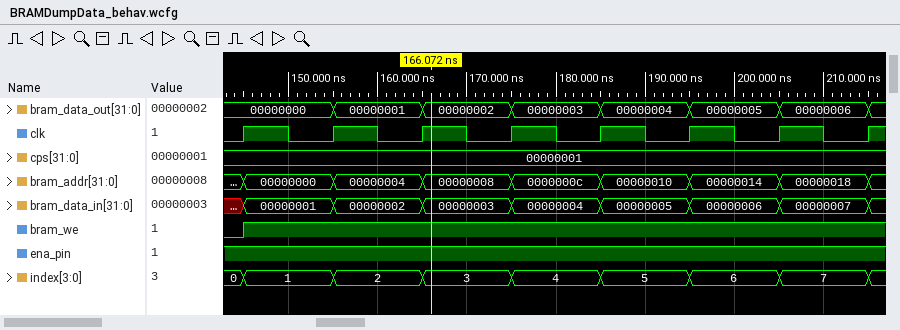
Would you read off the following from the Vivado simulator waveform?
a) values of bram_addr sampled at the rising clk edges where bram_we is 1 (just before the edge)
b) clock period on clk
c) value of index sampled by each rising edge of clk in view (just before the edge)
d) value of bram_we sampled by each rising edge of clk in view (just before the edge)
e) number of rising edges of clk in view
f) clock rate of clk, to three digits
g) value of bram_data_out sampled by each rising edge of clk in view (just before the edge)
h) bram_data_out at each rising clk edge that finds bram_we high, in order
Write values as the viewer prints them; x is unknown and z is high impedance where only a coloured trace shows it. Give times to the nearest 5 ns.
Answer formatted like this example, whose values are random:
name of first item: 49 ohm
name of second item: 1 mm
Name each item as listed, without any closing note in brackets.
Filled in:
values of bram_addr sampled at the rising clk edges where bram_we is 1: 00000000, 00000004, 00000008, 0000000c, 00000010, 00000014, 00000018
clock period on clk: 10 ns
value of index sampled by each rising edge of clk in view: 0, 1, 2, 3, 4, 5, 6, 7
value of bram_we sampled by each rising edge of clk in view: 0 1 1 1 1 1 1 1
number of rising edges of clk in view: 8
clock rate of clk, to three digits: 100 MHz
value of bram_data_out sampled by each rising edge of clk in view: 00000000, 00000000, 00000001, 00000002, 00000003, 00000004, 00000005, 00000006
bram_data_out at each rising clk edge that finds bram_we high, in order: 00000000, 00000001, 00000002, 00000003, 00000004, 00000005, 00000006
